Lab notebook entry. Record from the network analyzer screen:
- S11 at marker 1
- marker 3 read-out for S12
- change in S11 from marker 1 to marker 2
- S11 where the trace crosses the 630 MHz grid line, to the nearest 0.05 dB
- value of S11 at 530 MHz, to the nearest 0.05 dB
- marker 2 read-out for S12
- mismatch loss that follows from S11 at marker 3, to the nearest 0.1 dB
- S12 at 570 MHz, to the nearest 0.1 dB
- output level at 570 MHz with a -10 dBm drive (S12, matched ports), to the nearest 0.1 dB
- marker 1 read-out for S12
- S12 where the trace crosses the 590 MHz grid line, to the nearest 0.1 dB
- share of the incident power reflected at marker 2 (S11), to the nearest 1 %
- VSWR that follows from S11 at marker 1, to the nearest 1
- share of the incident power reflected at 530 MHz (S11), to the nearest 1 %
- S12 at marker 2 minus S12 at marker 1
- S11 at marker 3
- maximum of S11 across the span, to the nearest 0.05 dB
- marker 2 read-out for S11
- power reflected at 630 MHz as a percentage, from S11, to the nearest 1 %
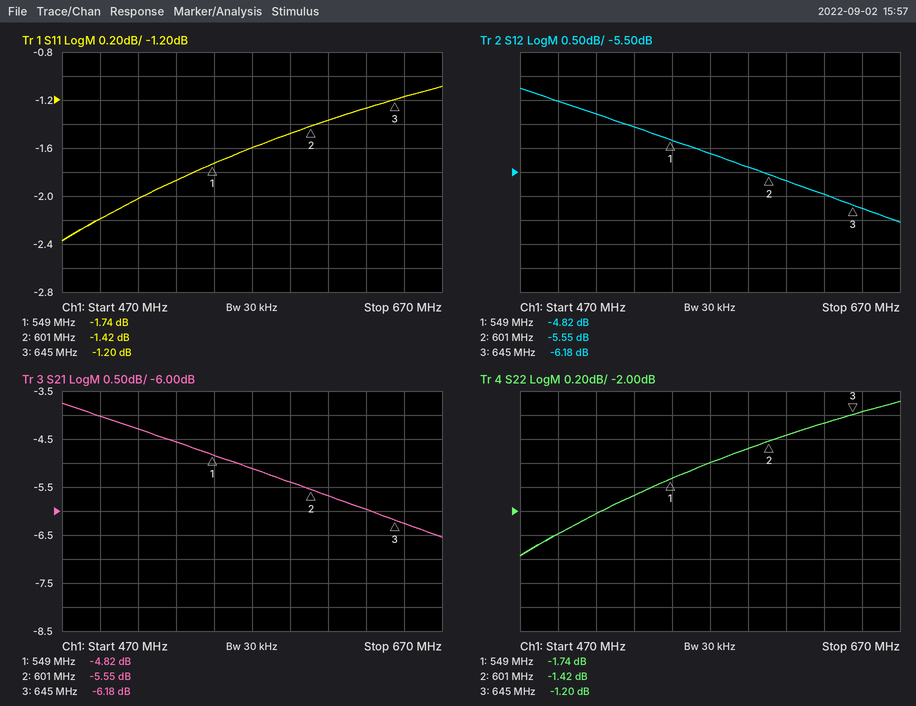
-1.74 dB
-6.18 dB
0.32 dB
-1.25 dB
-1.85 dB
-5.55 dB
6.2 dB
-5.1 dB
-15.1 dBm
-4.82 dB
-5.4 dB
72 %
10
65 %
-0.73 dB
-1.20 dB
-1.10 dB
-1.42 dB
75 %
